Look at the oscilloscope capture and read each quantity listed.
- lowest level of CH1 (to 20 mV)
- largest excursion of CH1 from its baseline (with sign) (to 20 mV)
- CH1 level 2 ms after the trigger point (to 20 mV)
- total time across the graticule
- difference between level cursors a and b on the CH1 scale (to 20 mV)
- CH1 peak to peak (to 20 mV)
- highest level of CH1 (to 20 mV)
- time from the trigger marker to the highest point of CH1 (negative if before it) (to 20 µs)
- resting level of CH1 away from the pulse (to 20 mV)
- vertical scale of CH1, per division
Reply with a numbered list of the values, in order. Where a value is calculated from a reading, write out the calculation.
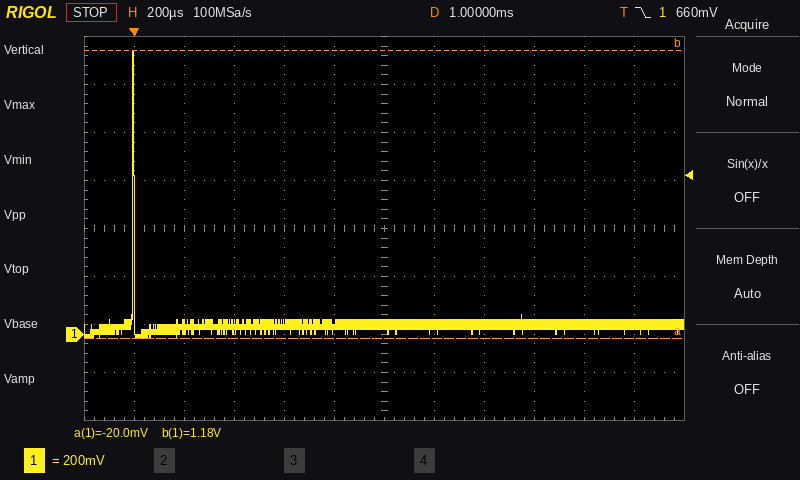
1. -20 mV
2. 1.18 V − (40 mV) = +1.14 V
3. 40 mV
4. 2.4 ms
5. 1.20 V
6. 1.18 V − (-20 mV) = 1.20 V
7. 1.18 V
8. 0 µs
9. 40 mV
10. 200 mV
